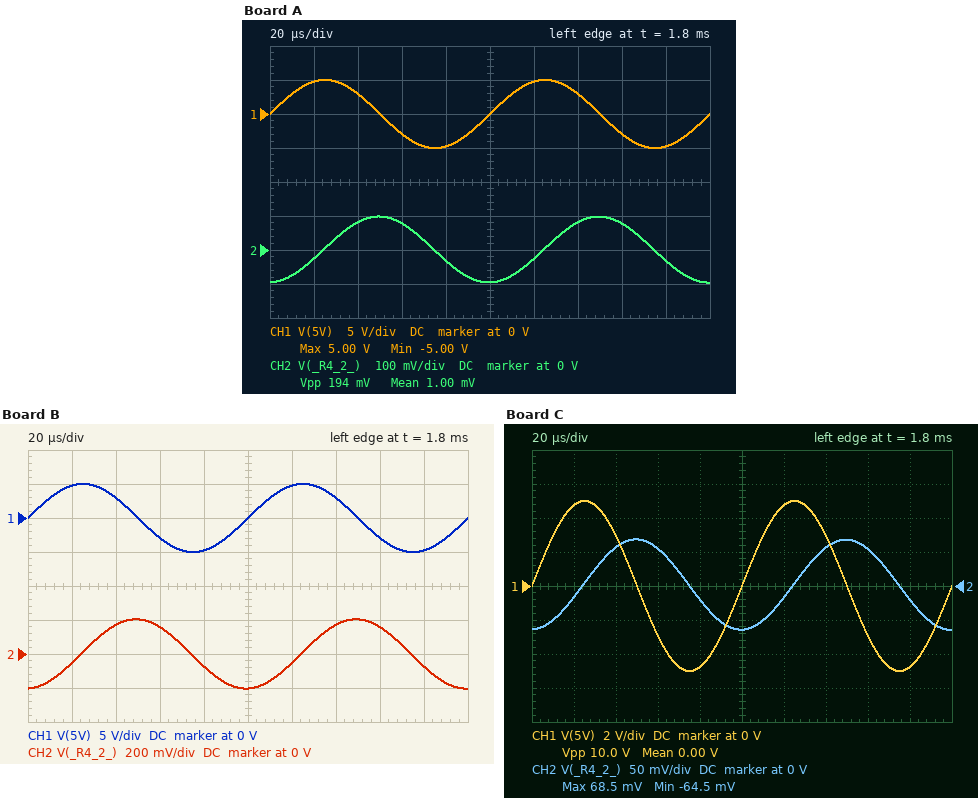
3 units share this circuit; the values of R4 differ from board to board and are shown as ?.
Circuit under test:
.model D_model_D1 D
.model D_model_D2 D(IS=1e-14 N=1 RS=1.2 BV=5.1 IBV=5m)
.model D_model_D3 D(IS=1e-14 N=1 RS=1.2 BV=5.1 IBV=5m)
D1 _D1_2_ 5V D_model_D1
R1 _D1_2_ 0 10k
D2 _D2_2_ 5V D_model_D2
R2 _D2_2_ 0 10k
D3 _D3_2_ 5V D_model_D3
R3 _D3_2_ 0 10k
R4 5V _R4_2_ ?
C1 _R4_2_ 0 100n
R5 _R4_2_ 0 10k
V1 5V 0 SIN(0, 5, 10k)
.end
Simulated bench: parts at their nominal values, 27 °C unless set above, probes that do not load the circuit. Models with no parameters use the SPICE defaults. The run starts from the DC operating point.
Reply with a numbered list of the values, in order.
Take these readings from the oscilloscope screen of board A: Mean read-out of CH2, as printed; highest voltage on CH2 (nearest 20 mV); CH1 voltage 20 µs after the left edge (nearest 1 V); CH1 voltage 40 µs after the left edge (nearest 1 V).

1. 1.00 mV
2. 100 mV
3. 5 V
4. 3 V
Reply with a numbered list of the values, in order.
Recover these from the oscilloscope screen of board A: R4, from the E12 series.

1. 8.2 kΩ
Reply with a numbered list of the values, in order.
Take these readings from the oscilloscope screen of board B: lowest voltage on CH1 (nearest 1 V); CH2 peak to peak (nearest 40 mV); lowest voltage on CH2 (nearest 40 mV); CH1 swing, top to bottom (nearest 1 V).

1. -5 V
2. 400 mV
3. -200 mV
4. 10 V
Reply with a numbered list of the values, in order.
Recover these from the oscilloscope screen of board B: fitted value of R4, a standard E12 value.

1. 3.9 kΩ
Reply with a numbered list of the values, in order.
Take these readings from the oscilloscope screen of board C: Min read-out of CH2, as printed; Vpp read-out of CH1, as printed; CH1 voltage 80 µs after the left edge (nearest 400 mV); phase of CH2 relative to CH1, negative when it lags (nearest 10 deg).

1. -64.5 mV
2. 10.0 V
3. -4.8 V
4. -90 deg
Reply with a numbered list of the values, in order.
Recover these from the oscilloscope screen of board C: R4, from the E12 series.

1. 12 kΩ
